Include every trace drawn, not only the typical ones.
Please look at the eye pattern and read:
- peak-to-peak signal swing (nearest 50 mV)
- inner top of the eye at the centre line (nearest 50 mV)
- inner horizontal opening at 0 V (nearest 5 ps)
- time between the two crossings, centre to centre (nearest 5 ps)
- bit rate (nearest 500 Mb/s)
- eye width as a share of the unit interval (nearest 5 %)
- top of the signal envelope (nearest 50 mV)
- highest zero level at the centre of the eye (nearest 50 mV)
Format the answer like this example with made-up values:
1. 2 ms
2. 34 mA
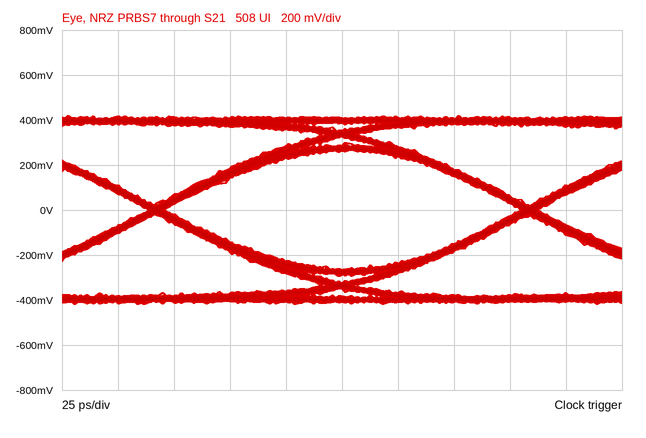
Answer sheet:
1. 850 mV
2. 250 mV
3. 160 ps
4. 165 ps
5. 6.0 Gb/s
6. 95 %
7. 400 mV
8. -250 mV
